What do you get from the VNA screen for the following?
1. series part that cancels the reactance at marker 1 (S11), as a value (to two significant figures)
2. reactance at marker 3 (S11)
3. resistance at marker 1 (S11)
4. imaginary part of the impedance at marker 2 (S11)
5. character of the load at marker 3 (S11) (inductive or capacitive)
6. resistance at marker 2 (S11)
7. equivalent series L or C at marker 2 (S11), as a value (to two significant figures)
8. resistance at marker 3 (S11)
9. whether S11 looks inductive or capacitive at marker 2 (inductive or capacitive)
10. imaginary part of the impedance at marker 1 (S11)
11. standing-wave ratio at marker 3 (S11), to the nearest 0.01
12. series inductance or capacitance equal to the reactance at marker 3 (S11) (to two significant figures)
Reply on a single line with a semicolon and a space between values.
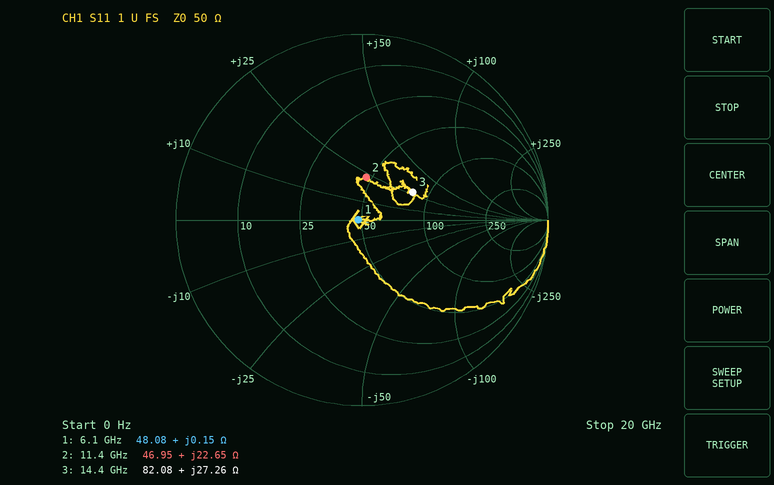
170 pF; +27.26 Ω; 48.08 Ω; +22.65 Ω; inductive; 46.95 Ω; 320 pH; 82.08 Ω; inductive; +0.15 Ω; 1.91; 300 pH
